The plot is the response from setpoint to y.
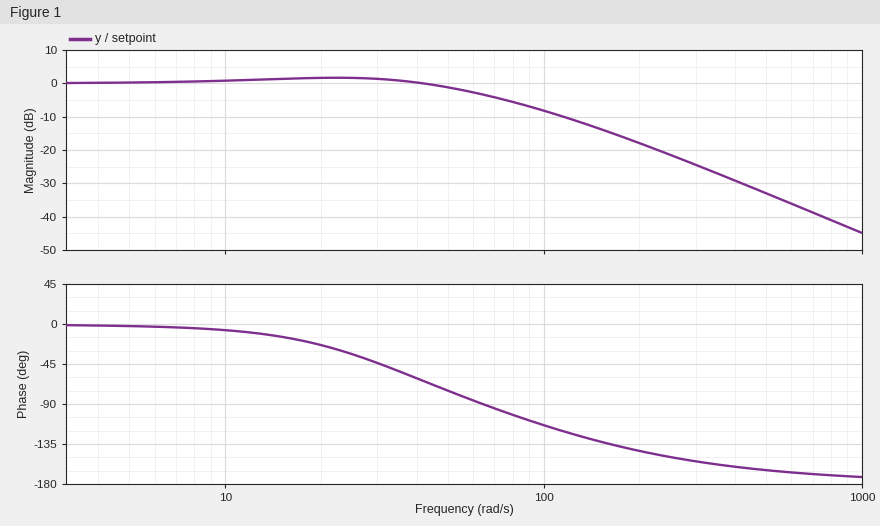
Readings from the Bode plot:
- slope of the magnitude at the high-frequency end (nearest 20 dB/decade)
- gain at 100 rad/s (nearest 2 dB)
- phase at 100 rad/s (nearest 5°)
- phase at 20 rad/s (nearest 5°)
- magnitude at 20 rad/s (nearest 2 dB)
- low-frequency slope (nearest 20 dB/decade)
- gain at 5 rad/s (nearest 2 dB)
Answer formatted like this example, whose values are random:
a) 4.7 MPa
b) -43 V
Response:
a) -40 dB/decade
b) -8 dB
c) -115°
d) -25°
e) 2 dB
f) 0 dB/decade
g) 0 dB
